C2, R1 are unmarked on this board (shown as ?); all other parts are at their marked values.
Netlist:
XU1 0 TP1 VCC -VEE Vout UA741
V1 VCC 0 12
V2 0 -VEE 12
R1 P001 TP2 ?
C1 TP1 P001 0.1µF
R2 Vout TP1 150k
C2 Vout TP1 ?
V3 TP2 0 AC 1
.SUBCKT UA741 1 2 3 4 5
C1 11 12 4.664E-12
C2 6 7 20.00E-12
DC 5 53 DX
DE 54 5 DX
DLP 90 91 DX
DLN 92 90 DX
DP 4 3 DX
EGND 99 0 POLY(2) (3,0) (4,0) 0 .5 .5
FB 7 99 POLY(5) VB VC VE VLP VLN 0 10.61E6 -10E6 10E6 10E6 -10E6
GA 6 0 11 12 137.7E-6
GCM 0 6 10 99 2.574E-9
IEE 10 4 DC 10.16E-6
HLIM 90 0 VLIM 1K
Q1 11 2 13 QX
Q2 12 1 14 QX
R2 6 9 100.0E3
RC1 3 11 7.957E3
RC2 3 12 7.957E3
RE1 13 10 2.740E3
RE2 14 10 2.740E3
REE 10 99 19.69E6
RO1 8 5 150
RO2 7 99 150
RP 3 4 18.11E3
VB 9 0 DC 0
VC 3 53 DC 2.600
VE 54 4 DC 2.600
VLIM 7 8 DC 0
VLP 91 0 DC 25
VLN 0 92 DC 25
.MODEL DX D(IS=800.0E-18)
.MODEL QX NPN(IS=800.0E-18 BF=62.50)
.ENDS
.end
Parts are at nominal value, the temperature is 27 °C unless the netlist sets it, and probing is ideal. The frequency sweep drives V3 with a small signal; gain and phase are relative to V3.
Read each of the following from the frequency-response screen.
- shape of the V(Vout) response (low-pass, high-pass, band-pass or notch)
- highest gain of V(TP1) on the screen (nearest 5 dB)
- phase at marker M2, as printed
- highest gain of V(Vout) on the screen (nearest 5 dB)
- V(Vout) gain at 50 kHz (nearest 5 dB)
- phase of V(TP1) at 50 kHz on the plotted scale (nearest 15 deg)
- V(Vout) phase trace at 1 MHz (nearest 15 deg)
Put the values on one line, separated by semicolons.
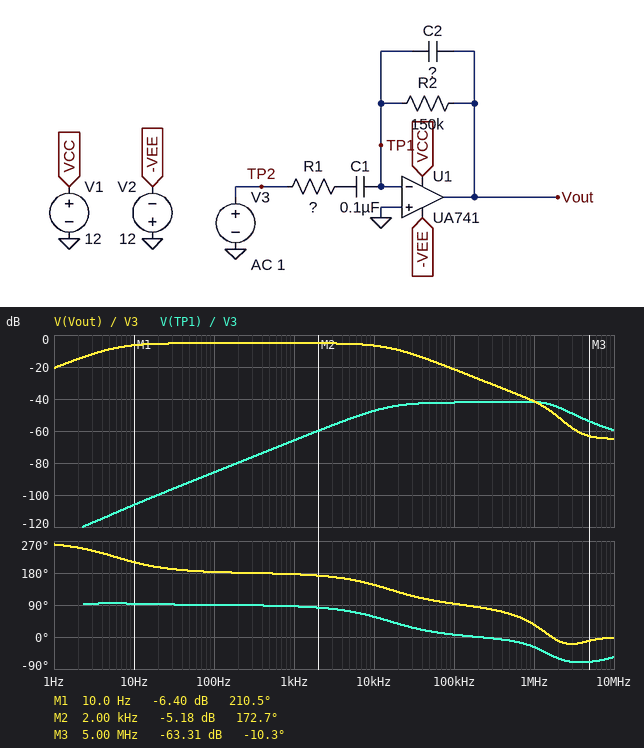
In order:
band-pass; -40 dB; 172.7 deg; -5 dB; -15 dB; 15 deg; 30 deg
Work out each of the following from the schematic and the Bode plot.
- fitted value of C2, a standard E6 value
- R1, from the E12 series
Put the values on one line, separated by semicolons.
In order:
68 pF; 270 kΩ
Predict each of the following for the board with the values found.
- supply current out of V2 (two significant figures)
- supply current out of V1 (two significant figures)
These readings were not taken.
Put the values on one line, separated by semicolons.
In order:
1.3 mA; 1.3 mA
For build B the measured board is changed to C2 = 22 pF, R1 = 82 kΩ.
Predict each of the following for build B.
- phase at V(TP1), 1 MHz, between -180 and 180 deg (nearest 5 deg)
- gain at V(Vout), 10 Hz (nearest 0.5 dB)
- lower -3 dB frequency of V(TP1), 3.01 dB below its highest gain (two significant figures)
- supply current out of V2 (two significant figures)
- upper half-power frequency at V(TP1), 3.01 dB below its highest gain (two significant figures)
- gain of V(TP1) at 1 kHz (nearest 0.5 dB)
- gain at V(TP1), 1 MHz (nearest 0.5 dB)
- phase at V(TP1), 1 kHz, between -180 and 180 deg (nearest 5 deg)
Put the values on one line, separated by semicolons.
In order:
-25 deg; -1.5 dB; 48 kHz; 1.3 mA; 2.0 MHz; -55.5 dB; -22.5 dB; 90 deg
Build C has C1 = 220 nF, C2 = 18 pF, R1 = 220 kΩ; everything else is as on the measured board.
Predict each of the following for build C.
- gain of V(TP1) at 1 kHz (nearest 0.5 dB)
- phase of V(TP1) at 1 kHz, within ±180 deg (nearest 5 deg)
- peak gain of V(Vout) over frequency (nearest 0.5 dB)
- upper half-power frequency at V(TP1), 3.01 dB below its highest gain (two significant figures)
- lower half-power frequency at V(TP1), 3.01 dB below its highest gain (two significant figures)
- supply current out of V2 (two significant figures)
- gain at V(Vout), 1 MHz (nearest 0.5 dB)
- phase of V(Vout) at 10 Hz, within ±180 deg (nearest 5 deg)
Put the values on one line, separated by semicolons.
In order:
-64.0 dB; 90 deg; -3.5 dB; 2.0 MHz; 60 kHz; 1.3 mA; -29.0 dB; -160 deg
